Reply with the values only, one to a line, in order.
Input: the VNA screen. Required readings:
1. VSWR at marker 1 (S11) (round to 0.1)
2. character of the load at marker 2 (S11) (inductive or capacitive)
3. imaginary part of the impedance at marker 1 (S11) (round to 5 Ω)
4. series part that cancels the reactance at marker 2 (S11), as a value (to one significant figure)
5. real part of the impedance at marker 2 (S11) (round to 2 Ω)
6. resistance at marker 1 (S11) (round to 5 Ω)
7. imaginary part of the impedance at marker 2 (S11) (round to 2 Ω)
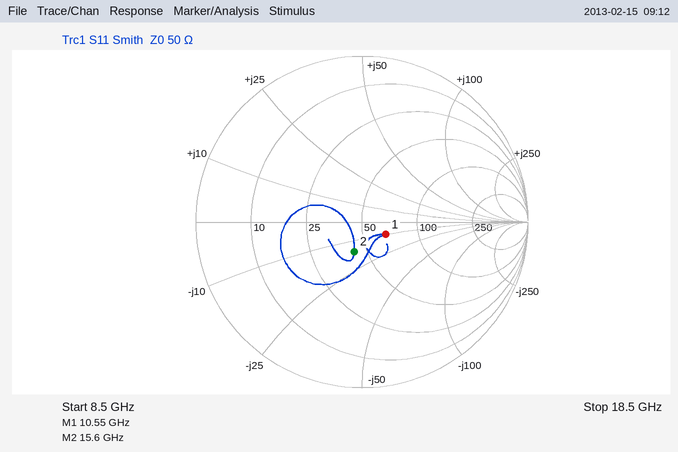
1.4
capacitive
-10 Ω
200 pH
42 Ω
65 Ω
-16 Ω
